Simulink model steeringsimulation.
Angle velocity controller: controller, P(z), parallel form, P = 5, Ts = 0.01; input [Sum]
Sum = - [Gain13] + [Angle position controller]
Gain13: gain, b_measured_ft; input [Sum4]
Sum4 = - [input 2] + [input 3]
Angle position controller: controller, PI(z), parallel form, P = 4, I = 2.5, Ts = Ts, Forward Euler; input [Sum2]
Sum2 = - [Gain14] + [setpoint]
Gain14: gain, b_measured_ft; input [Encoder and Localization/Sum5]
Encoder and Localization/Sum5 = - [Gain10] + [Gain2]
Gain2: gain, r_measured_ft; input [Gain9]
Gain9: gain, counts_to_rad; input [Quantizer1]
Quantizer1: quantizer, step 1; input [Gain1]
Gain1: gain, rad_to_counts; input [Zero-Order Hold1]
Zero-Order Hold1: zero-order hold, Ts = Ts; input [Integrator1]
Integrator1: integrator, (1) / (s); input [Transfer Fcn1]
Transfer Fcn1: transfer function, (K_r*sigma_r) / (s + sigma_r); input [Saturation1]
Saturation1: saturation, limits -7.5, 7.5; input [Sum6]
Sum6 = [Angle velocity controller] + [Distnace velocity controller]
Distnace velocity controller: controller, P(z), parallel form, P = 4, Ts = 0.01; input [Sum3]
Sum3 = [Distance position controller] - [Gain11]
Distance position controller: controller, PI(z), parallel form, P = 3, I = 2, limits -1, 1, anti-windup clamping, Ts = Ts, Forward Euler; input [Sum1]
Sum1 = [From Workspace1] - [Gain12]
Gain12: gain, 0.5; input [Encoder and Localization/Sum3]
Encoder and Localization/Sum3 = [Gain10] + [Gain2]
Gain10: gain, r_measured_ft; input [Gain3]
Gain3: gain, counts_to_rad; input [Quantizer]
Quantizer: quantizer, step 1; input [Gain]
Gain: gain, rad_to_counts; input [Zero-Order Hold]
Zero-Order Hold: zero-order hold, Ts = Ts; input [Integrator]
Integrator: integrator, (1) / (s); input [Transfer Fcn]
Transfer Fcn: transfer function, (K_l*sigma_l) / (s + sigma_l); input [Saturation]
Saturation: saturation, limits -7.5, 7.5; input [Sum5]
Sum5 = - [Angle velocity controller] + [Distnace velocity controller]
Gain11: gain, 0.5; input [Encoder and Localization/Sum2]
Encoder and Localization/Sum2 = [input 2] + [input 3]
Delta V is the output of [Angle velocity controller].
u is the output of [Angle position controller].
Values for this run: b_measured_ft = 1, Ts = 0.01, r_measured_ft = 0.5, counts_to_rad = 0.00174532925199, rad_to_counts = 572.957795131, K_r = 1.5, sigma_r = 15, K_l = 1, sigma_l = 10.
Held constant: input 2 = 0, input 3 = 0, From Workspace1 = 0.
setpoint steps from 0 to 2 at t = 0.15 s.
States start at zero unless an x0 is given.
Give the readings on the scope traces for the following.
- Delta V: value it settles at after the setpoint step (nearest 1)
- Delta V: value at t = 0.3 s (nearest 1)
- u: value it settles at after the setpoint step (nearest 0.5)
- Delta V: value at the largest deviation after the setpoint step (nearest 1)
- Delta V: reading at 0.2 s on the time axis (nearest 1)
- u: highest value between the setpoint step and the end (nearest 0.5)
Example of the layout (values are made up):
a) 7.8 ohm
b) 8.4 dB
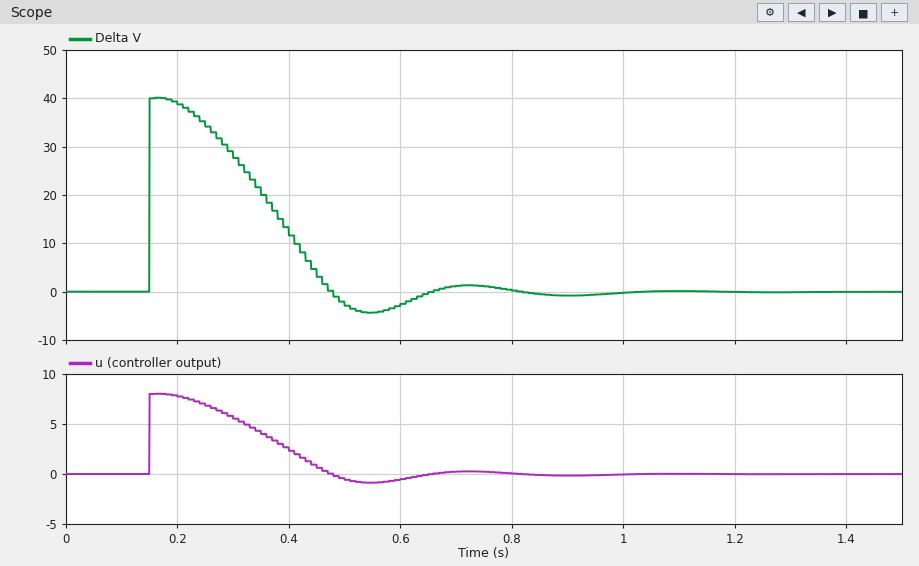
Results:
a) 0
b) 28
c) 0.0
d) 40
e) 39
f) 8.0
